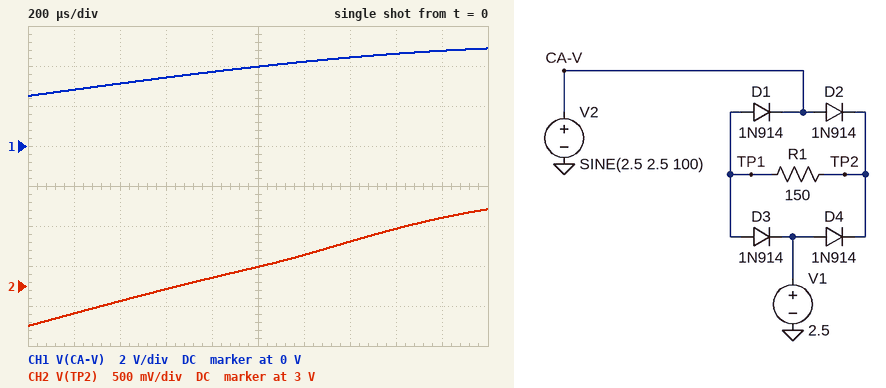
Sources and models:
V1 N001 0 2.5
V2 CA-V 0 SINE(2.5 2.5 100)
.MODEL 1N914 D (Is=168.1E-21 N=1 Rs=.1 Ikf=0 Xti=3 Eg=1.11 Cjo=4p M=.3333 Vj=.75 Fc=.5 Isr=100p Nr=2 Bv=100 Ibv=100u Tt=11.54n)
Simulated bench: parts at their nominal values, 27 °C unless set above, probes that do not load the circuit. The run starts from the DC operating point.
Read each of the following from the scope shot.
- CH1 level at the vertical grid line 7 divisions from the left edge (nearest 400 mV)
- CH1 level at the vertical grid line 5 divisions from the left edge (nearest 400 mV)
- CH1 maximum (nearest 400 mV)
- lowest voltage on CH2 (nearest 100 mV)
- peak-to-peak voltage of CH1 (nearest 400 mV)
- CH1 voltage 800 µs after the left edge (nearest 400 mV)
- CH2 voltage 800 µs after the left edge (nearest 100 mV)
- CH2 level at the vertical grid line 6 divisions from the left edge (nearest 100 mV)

4.4 V
4.0 V
4.8 V
2.5 V
2.4 V
3.6 V
3.1 V
3.4 V
